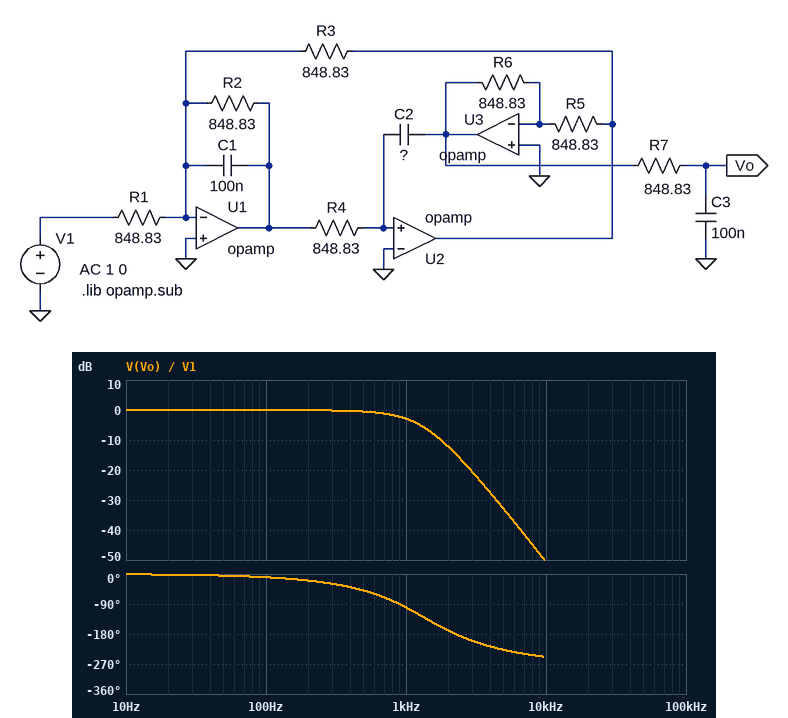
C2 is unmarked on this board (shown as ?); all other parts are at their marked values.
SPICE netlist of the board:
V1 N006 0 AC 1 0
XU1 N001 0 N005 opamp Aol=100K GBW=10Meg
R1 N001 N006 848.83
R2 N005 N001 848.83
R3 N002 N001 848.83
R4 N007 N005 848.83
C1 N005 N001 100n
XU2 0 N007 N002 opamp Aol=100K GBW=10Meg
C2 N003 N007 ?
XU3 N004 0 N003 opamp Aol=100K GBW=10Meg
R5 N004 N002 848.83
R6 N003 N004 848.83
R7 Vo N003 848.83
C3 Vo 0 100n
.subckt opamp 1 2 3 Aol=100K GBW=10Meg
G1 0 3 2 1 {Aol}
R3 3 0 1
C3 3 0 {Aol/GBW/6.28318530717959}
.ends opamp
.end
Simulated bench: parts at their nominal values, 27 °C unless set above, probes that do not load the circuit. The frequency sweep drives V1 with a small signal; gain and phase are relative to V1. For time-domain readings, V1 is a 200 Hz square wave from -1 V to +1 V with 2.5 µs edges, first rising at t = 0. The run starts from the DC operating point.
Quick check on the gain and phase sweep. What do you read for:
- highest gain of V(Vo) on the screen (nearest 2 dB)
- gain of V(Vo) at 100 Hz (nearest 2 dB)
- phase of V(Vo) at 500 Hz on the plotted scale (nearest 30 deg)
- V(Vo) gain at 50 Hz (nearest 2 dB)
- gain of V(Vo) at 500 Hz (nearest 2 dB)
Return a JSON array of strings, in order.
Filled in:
["0 dB", "0 dB", "-60 deg", "0 dB", "0 dB"]
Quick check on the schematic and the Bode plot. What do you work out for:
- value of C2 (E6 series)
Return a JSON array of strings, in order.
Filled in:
["220 nF"]
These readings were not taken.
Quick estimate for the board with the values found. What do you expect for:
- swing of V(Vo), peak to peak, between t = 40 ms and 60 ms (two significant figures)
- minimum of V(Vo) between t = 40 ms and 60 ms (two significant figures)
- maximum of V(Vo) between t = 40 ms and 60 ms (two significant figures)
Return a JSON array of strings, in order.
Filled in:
["2.1 V", "-1.0 V", "1.0 V"]
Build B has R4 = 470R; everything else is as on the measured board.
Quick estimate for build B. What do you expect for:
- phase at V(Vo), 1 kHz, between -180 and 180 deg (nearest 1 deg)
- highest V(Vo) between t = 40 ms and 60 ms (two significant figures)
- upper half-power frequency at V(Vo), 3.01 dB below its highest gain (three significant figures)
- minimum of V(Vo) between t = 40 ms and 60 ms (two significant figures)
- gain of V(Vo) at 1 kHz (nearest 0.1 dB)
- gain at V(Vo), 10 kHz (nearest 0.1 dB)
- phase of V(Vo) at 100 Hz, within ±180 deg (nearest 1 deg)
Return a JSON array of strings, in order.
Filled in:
["-73 deg", "1.1 V", "1.64 kHz", "-1.1 V", "-0.4 dB", "-45.4 dB", "-7 deg"]
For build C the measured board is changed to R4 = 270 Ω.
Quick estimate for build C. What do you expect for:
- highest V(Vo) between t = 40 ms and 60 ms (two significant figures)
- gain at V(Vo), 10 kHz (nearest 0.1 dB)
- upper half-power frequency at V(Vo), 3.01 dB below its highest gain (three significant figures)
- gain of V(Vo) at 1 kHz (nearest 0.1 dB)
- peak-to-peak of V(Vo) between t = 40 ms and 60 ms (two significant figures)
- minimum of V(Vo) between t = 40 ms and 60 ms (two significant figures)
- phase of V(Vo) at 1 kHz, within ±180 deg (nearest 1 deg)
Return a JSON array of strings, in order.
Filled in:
["1.2 V", "-40.4 dB", "2.35 kHz", "0 dB", "2.4 V", "-1.2 V", "-53 deg"]
